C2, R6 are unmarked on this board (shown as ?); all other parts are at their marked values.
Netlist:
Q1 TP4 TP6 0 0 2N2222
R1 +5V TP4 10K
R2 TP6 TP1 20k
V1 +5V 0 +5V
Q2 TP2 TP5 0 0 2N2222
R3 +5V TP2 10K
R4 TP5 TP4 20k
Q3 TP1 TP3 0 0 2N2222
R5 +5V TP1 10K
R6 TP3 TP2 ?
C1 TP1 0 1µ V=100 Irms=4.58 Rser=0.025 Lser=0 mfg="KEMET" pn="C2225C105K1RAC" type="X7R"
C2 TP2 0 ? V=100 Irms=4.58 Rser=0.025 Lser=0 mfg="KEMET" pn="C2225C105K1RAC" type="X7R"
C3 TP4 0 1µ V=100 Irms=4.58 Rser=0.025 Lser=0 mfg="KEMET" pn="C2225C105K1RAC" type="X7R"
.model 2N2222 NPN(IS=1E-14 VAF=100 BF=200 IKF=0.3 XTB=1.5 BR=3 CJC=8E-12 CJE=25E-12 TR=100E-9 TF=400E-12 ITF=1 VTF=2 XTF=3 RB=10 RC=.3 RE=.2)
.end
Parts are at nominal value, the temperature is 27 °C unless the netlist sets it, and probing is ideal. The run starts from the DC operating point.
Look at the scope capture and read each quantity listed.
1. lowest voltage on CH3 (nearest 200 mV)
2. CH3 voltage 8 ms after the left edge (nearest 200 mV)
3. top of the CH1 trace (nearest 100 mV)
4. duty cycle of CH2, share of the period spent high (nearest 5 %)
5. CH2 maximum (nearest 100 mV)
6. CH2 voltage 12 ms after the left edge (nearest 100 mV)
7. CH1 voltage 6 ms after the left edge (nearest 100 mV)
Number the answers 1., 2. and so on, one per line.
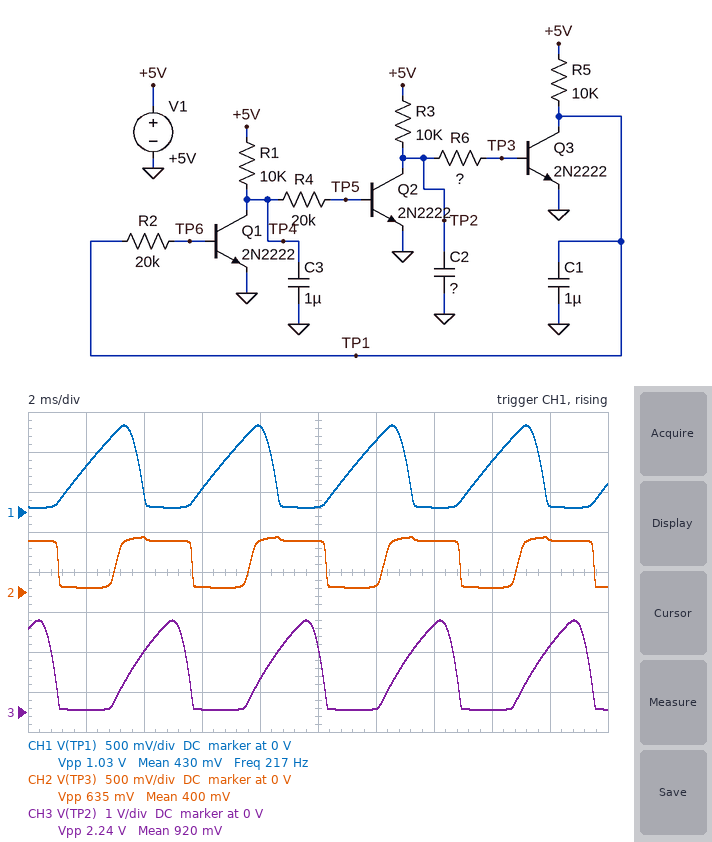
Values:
1. 0 V
2. 800 mV
3. 1.1 V
4. 55 %
5. 700 mV
6. 100 mV
7. 300 mV
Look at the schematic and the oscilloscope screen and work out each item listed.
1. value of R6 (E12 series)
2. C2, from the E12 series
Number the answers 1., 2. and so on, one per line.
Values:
1. 56 kΩ
2. 330 nF
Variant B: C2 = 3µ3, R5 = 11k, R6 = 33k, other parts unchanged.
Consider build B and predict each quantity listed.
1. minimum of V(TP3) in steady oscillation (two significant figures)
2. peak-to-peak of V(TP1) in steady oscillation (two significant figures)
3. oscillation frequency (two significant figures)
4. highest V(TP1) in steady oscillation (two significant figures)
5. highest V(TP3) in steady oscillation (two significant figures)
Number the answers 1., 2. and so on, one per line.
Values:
1. 46 mV
2. 1.9 V
3. 95 Hz
4. 2.0 V
5. 670 mV
